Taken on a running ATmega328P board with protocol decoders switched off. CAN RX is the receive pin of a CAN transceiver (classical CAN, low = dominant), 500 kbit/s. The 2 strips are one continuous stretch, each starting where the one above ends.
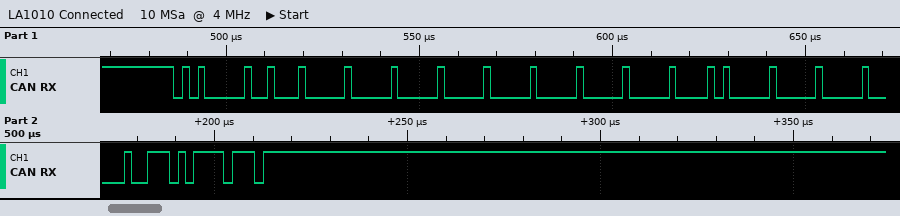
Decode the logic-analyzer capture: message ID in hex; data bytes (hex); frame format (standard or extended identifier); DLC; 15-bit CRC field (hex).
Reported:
0x501
00 00 00 00 00 50 00 00
standard
8
0x1D7B
